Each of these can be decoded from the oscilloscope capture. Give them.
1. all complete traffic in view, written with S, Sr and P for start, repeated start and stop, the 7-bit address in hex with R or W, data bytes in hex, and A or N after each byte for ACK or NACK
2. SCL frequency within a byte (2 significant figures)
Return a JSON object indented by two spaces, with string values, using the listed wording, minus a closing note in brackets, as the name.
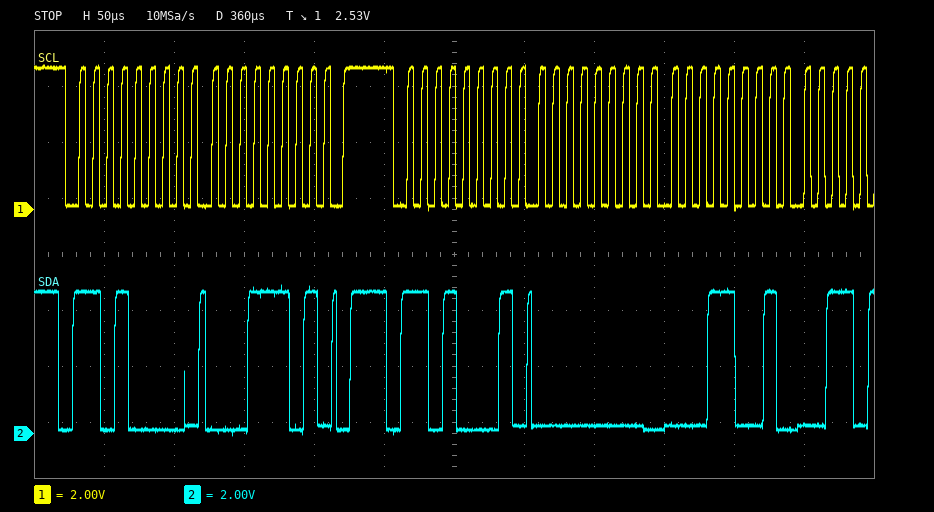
{
  "all complete traffic in view, written with S, Sr and P for start, repeated start and stop, the 7-bit address in hex with R or W, data bytes in hex, and A or N after each byte for ACK or NACK": "S 68W A 1D A P S 68R A 00 A 19 A",
  "SCL frequency within a byte": "100 kHz"
}
